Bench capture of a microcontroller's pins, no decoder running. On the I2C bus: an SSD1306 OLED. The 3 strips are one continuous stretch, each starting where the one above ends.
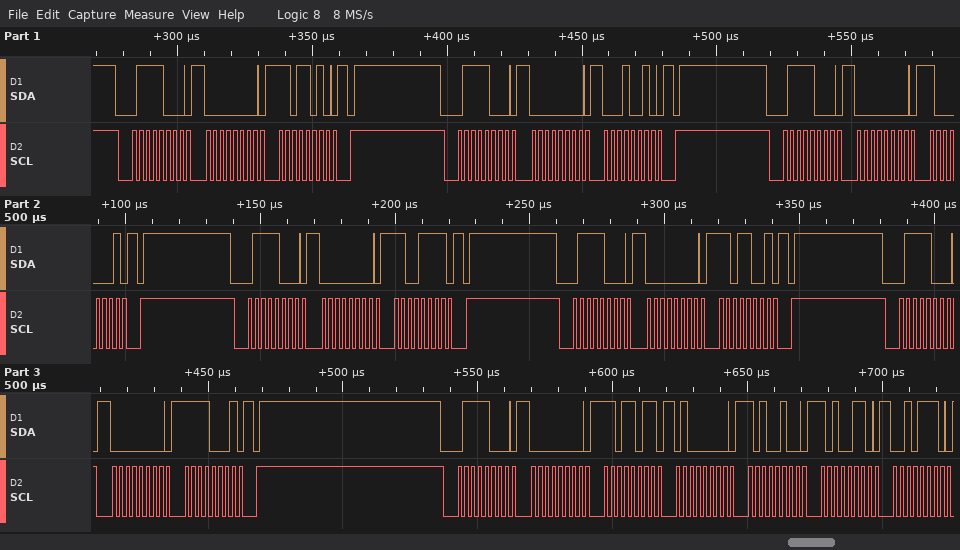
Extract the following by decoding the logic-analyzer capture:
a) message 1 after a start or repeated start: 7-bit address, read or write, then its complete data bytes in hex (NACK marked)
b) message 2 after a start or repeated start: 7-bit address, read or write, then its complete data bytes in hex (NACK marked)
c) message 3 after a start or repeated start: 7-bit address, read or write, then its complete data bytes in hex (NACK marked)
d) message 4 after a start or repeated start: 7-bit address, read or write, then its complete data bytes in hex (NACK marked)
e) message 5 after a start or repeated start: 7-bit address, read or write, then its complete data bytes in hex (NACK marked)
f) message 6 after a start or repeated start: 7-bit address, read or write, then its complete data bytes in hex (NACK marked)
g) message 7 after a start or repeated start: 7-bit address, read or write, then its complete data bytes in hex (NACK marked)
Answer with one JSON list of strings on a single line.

["0x3C write: 00 DA", "0x3C write: 00 12", "0x3C write: 00 81", "0x3C write: 00 CF", "0x3C write: 00 D9", "0x3C write: 00 F1", "0x3C write: 00 DB 40 A4 A6 2E"]
